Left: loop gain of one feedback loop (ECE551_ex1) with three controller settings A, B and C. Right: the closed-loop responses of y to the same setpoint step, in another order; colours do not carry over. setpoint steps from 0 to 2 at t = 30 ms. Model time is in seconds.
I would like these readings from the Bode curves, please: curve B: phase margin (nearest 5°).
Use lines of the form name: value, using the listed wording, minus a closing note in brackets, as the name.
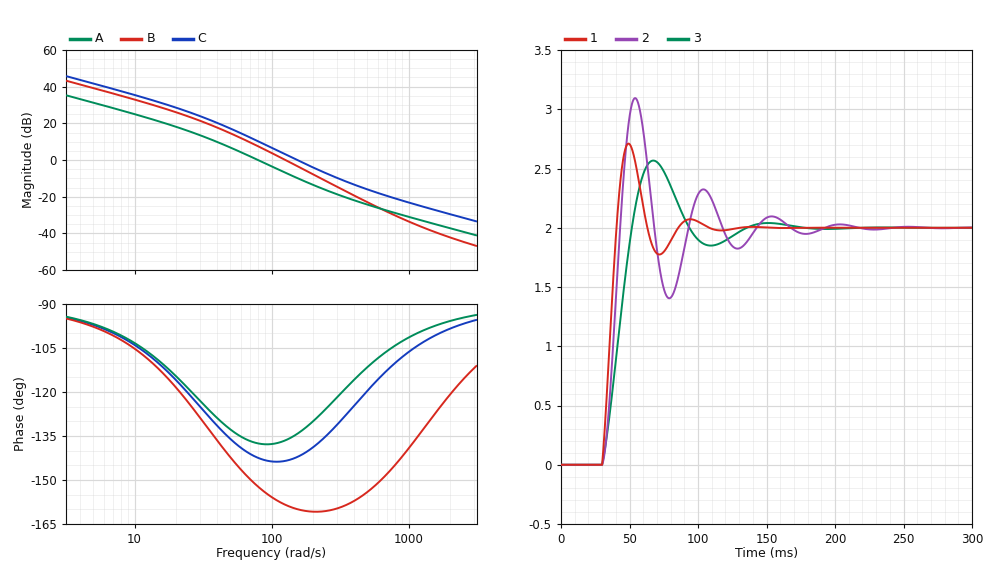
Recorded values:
curve B: phase margin: 20°
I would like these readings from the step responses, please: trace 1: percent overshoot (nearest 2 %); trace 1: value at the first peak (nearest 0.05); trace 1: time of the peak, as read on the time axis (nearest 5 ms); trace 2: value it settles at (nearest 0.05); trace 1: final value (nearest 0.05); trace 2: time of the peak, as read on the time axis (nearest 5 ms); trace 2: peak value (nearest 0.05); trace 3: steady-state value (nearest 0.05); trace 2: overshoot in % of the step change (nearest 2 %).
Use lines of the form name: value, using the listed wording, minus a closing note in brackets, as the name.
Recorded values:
trace 1: percent overshoot: 36 %
trace 1: value at the first peak: 2.70
trace 1: time of the peak, as read on the time axis: 50 ms
trace 2: value it settles at: 2.00
trace 1: final value: 2.00
trace 2: time of the peak, as read on the time axis: 55 ms
trace 2: peak value: 3.10
trace 3: steady-state value: 2.00
trace 2: overshoot in % of the step change: 54 %
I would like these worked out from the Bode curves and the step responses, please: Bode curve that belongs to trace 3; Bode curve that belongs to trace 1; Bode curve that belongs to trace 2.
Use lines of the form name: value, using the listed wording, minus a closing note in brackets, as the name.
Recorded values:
Bode curve that belongs to trace 3: A
Bode curve that belongs to trace 1: C
Bode curve that belongs to trace 2: B
